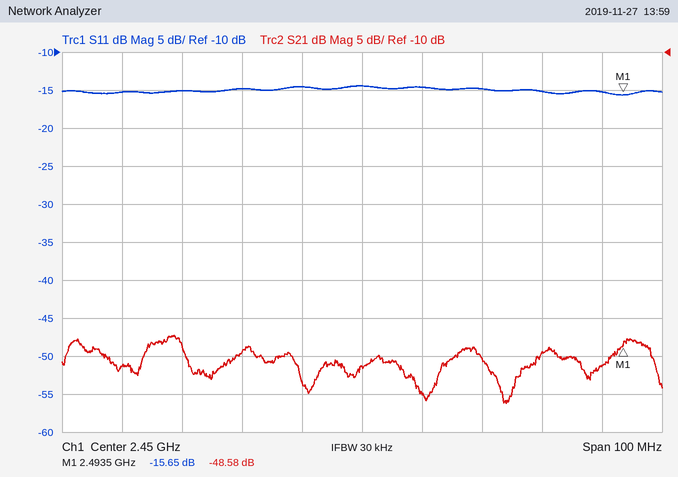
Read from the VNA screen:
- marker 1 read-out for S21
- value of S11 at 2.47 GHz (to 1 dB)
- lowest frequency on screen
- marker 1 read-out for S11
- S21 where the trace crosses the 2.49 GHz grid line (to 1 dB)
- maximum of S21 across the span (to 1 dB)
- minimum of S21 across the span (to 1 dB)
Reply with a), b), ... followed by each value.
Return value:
a) -48.58 dB
b) -15 dB
c) 2.4 GHz
d) -15.65 dB
e) -51 dB
f) -47 dB
g) -56 dB
